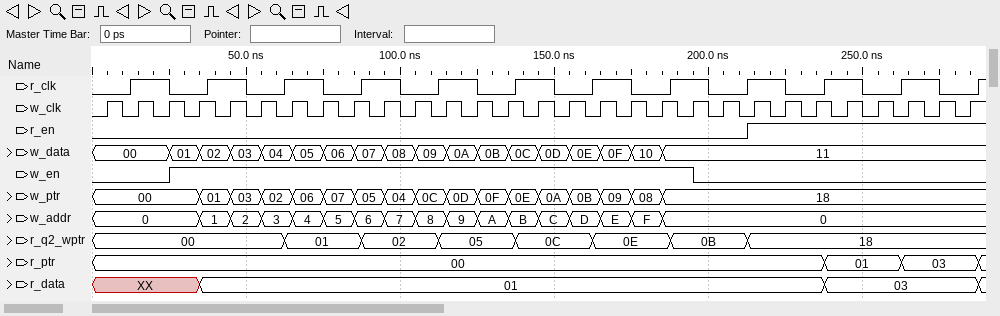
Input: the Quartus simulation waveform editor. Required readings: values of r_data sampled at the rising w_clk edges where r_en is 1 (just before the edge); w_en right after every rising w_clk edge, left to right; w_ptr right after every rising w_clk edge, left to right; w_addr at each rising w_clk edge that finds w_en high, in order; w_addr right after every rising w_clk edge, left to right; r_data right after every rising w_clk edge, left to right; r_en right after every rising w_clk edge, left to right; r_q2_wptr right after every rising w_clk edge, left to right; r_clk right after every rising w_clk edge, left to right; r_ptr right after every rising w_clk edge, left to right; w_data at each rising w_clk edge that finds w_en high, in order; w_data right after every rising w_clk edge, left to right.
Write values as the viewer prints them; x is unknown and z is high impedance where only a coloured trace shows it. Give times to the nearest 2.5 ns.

01, 01, 01, 03, 03, 03, 03, 03
0 0 1 1 1 1 1 1 1 1 1 1 1 1 1 1 1 1 1 0 0 0 0 0 0 0 0 0 0
00, 00, 00, 01, 03, 02, 06, 07, 05, 04, 0C, 0D, 0F, 0E, 0A, 0B, 09, 08, 18, 18, 18, 18, 18, 18, 18, 18, 18, 18, 18
0, 1, 2, 3, 4, 5, 6, 7, 8, 9, A, B, C, D, E, F, 0
0, 0, 0, 1, 2, 3, 4, 5, 6, 7, 8, 9, A, B, C, D, E, F, 0, 0, 0, 0, 0, 0, 0, 0, 0, 0, 0
XX, XX, XX, 01, 01, 01, 01, 01, 01, 01, 01, 01, 01, 01, 01, 01, 01, 01, 01, 01, 01, 01, 01, 01, 03, 03, 03, 03, 03
0 0 0 0 0 0 0 0 0 0 0 0 0 0 0 0 0 0 0 0 0 1 1 1 1 1 1 1 1
00, 00, 00, 00, 00, 00, 01, 01, 01, 02, 02, 05, 05, 05, 0C, 0C, 0E, 0E, 0E, 0B, 0B, 18, 18, 18, 18, 18, 18, 18, 18
0 1 0 0 1 0 1 0 0 1 0 1 0 0 1 0 1 0 0 1 0 1 0 0 1 0 1 0 0
00, 00, 00, 00, 00, 00, 00, 00, 00, 00, 00, 00, 00, 00, 00, 00, 00, 00, 00, 00, 00, 00, 00, 00, 01, 01, 03, 03, 03
01, 02, 03, 04, 05, 06, 07, 08, 09, 0A, 0B, 0C, 0D, 0E, 0F, 10, 11
00, 00, 01, 02, 03, 04, 05, 06, 07, 08, 09, 0A, 0B, 0C, 0D, 0E, 0F, 10, 11, 11, 11, 11, 11, 11, 11, 11, 11, 11, 11
